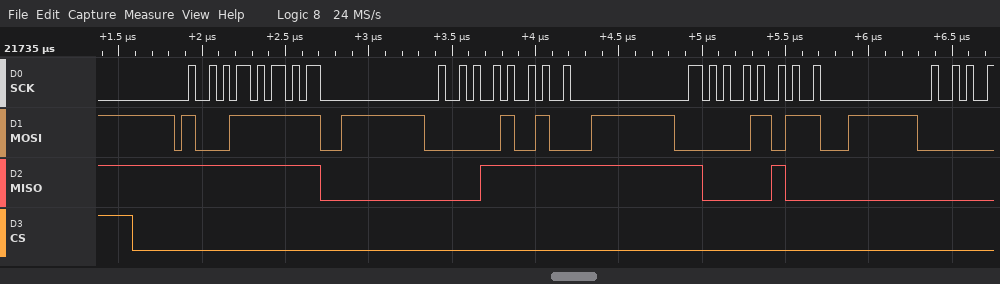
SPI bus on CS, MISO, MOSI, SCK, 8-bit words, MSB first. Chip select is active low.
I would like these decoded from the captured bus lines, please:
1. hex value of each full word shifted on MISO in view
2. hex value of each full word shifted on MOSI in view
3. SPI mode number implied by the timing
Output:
FF, 1F, 84
9F, 0A, 0B
0
